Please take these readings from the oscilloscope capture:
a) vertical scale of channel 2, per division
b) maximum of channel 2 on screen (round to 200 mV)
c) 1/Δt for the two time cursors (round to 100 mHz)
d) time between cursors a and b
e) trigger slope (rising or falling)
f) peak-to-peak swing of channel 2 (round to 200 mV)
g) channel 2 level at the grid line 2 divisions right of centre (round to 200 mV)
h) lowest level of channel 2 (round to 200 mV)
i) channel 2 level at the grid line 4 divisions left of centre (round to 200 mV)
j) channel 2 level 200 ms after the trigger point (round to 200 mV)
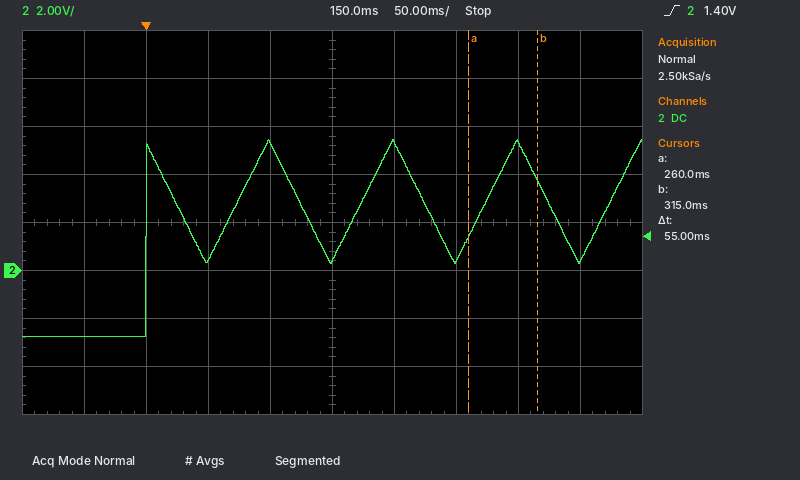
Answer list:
2 V
5.4 V
18.2 Hz
55 ms
rising
8.2 V
400 mV
-2.8 V
-2.8 V
5.2 V
